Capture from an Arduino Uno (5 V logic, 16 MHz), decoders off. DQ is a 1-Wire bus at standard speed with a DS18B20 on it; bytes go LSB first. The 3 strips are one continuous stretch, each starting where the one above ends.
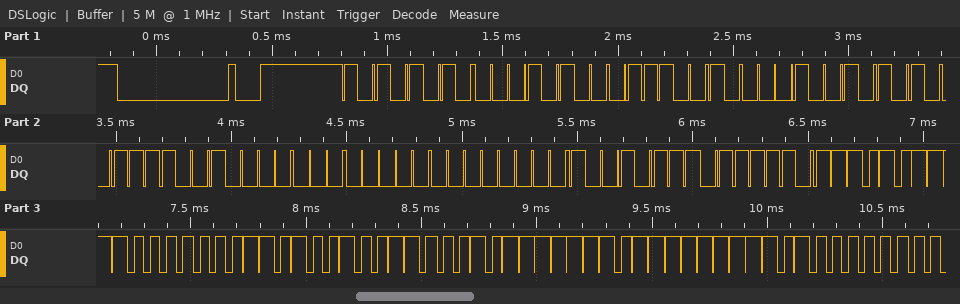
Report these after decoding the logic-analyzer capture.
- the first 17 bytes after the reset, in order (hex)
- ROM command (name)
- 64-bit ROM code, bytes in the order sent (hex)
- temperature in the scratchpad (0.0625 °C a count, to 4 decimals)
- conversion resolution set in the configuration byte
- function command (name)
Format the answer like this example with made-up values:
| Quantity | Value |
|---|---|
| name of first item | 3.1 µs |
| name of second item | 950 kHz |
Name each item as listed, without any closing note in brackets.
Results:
| Quantity | Value |
|---|---|
| the first 17 bytes after the reset, in order | 55 28 4E 48 E5 09 00 00 E9 BE EB 01 4B 46 7F FF 05 |
| ROM command | Match ROM |
| 64-bit ROM code, bytes in the order sent | 28 4E 48 E5 09 00 00 E9 |
| temperature in the scratchpad | 30.6875 °C |
| conversion resolution set in the configuration byte | 12 bits |
| function command | Read Scratchpad |
